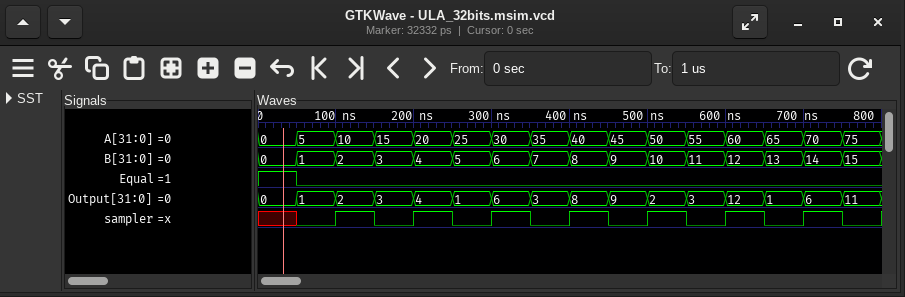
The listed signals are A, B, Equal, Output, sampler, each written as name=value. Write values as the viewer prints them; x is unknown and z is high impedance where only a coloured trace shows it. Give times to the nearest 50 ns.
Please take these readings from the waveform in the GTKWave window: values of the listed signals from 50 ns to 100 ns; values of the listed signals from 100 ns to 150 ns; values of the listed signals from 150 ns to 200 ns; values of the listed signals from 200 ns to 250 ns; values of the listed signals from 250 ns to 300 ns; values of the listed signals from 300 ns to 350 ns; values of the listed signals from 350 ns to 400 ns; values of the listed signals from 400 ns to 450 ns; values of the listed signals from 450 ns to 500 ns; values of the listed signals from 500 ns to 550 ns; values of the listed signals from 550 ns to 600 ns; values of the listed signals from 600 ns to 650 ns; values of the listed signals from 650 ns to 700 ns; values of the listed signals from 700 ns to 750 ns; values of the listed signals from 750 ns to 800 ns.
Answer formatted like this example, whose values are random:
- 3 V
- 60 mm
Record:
- A=5, B=1, Equal=0, Output=1, sampler=0
- A=10, B=2, Equal=0, Output=2, sampler=1
- A=15, B=3, Equal=0, Output=3, sampler=0
- A=20, B=4, Equal=0, Output=4, sampler=1
- A=25, B=5, Equal=0, Output=1, sampler=0
- A=30, B=6, Equal=0, Output=6, sampler=1
- A=35, B=7, Equal=0, Output=3, sampler=0
- A=40, B=8, Equal=0, Output=8, sampler=1
- A=45, B=9, Equal=0, Output=9, sampler=0
- A=50, B=10, Equal=0, Output=2, sampler=1
- A=55, B=11, Equal=0, Output=3, sampler=0
- A=60, B=12, Equal=0, Output=12, sampler=1
- A=65, B=13, Equal=0, Output=1, sampler=0
- A=70, B=14, Equal=0, Output=6, sampler=1
- A=75, B=15, Equal=0, Output=11, sampler=0
